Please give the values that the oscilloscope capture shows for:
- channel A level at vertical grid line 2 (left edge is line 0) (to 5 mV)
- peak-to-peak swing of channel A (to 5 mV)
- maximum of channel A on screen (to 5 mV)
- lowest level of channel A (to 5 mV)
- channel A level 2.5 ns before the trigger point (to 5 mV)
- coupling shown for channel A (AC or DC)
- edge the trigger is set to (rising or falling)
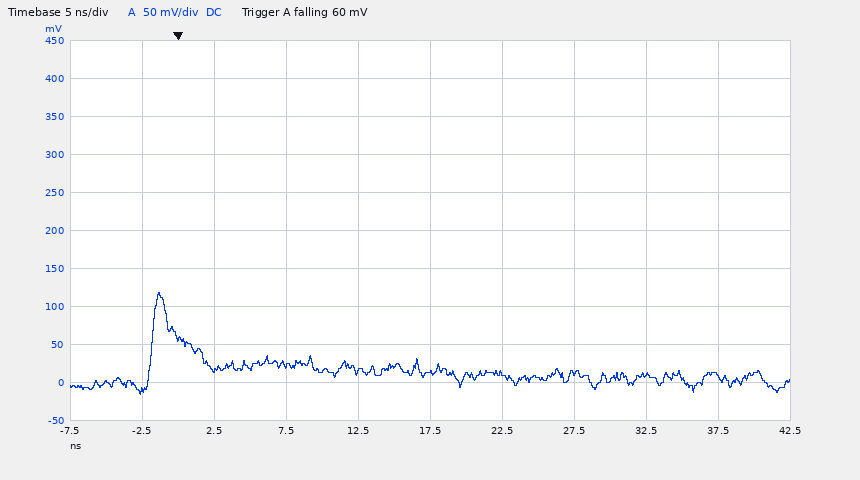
15 mV
135 mV
120 mV
-15 mV
-10 mV
DC
falling
